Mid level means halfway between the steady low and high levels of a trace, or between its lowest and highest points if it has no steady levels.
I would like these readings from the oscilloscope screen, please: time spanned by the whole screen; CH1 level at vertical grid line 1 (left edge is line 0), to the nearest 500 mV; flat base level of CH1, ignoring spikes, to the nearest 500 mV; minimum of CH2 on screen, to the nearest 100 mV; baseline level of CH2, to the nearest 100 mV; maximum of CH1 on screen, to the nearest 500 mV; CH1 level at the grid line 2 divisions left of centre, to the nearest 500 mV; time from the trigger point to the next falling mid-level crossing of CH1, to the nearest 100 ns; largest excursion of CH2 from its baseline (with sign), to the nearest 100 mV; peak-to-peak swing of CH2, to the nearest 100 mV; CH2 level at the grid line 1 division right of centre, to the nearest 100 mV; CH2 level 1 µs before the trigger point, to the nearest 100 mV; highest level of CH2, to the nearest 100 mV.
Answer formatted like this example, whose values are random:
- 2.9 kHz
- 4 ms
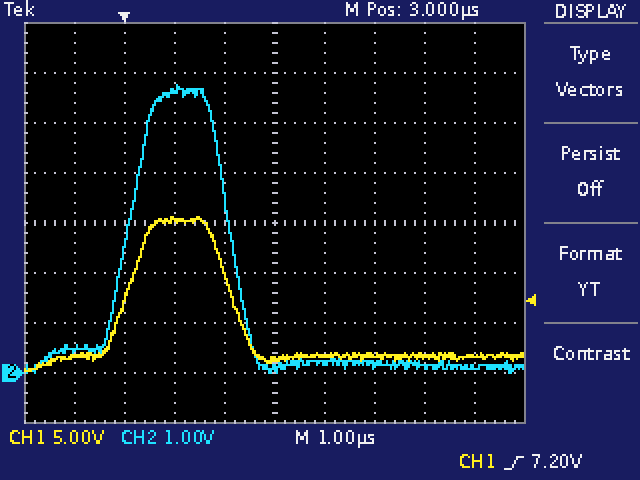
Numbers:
- 10 µs
- 1.5 V
- 1.5 V
- 0.0 V
- 200 mV
- 15.5 V
- 15.5 V
- 2.1 µs
- +5.6 V
- 5.8 V
- 200 mV
- 500 mV
- 5.8 V
